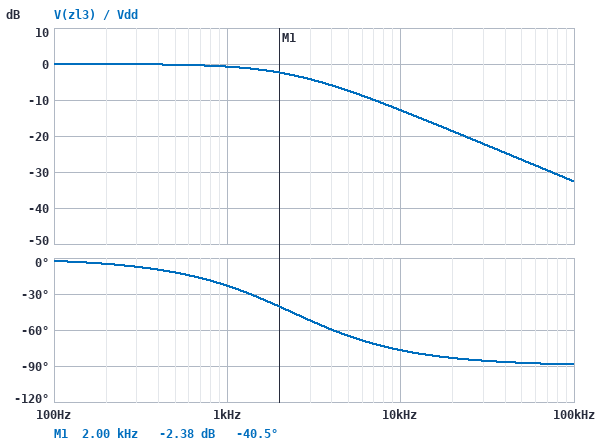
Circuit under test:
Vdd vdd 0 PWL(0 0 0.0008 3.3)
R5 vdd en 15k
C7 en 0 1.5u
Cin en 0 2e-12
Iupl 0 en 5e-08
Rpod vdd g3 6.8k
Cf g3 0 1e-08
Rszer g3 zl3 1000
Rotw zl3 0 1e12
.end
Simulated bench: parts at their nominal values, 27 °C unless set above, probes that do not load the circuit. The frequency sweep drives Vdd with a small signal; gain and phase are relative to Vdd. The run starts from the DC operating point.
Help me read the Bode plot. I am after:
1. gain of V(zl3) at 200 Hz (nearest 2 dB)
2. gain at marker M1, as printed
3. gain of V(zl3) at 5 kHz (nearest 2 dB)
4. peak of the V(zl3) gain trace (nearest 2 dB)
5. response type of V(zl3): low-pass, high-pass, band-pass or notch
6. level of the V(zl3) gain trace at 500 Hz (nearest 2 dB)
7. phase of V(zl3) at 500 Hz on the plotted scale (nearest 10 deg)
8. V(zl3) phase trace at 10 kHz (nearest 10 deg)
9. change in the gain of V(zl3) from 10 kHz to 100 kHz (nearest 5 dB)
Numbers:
0 dB
-2.38 dB
-8 dB
0 dB
low-pass
0 dB
-10 deg
-80 deg
-20 dB
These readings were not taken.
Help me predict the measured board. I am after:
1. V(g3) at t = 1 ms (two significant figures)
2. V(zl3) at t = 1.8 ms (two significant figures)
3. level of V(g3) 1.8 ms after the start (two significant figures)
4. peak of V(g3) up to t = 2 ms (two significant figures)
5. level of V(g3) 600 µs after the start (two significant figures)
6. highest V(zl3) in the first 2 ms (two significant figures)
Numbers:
3.3 V
3.3 V
3.3 V
3.3 V
2.2 V
3.3 V
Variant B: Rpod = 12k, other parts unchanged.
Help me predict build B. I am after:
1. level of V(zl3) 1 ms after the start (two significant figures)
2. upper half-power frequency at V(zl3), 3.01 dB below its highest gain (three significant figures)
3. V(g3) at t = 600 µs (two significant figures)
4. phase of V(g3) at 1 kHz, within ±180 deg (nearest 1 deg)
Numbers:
3.2 V
1.33 kHz
2.0 V
-37 deg
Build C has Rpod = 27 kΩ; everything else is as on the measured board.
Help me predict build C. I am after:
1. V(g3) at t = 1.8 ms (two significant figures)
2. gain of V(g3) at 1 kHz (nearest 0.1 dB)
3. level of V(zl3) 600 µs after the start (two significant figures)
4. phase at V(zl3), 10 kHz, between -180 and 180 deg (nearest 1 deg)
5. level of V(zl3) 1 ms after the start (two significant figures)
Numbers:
3.3 V
-5.9 dB
1.5 V
-87 deg
2.8 V
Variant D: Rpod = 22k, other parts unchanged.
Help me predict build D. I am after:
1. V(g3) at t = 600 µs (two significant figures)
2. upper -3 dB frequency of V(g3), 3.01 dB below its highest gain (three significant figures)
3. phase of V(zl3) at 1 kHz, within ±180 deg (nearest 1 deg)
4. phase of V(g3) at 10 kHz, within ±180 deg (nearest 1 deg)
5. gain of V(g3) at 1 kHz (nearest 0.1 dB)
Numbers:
1.6 V
723 Hz
-54 deg
-86 deg
-4.6 dB
